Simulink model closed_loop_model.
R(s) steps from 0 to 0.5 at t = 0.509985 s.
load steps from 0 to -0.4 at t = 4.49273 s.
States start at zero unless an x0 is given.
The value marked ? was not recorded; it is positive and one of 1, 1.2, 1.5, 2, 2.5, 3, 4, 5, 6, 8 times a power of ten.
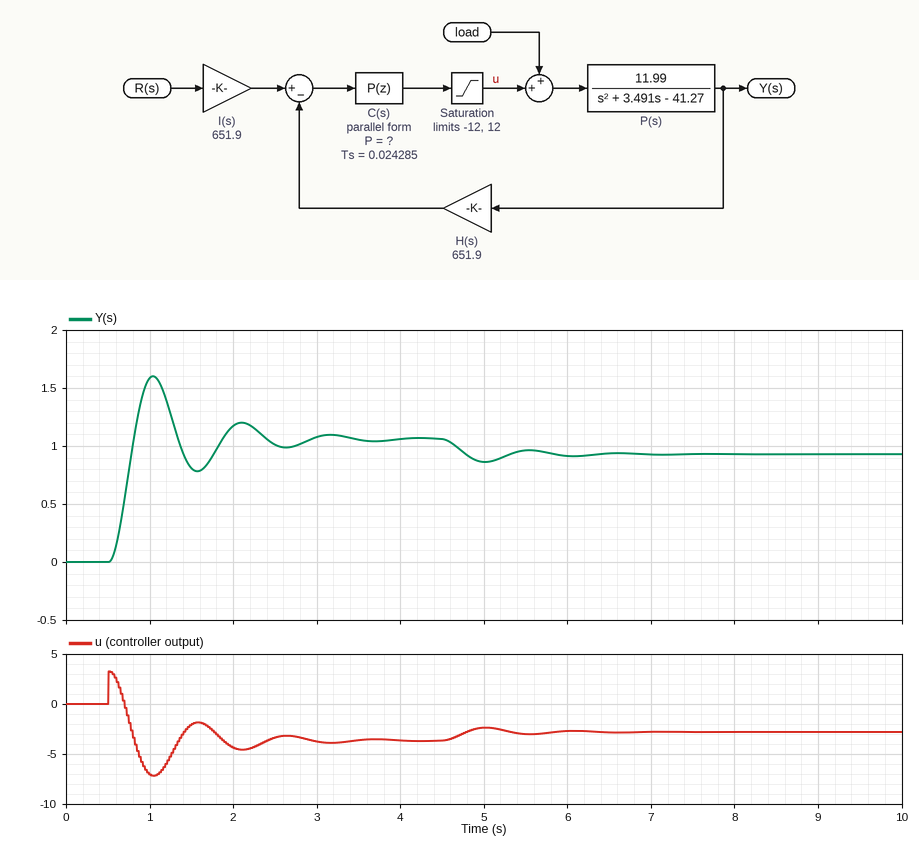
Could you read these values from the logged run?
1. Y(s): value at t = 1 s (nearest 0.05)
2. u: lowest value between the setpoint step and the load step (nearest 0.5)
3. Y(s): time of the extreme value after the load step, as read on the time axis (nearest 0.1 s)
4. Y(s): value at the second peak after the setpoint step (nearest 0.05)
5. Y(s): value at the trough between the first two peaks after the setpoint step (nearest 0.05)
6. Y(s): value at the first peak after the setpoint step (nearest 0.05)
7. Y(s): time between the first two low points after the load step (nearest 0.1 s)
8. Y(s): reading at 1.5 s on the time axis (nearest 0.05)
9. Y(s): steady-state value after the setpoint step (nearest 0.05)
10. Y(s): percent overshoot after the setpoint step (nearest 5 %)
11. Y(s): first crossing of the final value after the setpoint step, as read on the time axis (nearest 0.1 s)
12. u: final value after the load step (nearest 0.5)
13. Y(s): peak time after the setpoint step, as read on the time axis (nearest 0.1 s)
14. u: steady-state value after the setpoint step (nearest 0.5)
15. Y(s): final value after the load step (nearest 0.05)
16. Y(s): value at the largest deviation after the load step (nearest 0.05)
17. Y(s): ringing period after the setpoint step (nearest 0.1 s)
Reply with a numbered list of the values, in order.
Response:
1. 1.60
2. -7.0
3. 5.0 s
4. 1.20
5. 0.80
6. 1.60
7. 1.1 s
8. 0.80
9. 1.05
10. 50 %
11. 0.8 s
12. -3.0
13. 1.0 s
14. -3.5
15. 0.95
16. 0.85
17. 1.1 s
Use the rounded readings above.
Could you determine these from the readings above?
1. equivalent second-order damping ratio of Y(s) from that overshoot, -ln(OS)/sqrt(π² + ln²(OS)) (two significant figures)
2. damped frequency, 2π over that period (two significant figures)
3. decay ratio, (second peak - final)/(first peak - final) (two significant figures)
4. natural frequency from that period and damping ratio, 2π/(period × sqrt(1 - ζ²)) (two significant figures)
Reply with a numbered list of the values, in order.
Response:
1. 0.22
2. 5.7 rad/s
3. 0.27
4. 5.9 rad/s
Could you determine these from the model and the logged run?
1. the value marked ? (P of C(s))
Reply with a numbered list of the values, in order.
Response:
1. 0.01
